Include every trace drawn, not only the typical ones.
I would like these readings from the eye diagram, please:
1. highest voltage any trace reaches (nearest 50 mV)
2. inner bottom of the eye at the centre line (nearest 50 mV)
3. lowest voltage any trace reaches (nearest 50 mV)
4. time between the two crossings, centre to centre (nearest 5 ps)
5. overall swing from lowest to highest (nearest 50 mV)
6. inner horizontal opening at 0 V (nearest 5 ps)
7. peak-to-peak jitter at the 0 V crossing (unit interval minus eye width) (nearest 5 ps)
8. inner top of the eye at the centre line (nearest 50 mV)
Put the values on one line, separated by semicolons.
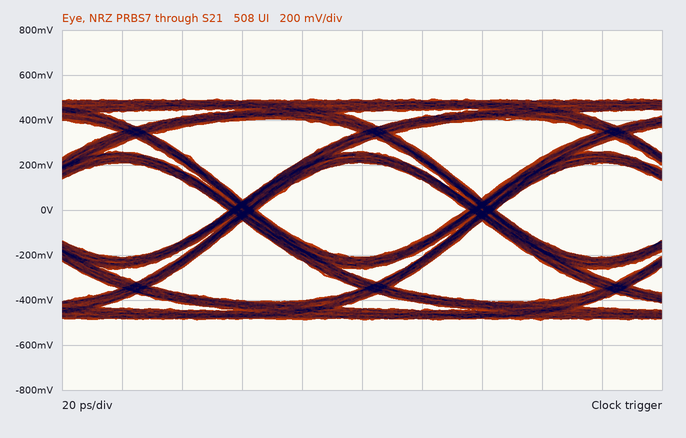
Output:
500 mV; -200 mV; -500 mV; 80 ps; 1.00 V; 70 ps; 10 ps; 200 mV
